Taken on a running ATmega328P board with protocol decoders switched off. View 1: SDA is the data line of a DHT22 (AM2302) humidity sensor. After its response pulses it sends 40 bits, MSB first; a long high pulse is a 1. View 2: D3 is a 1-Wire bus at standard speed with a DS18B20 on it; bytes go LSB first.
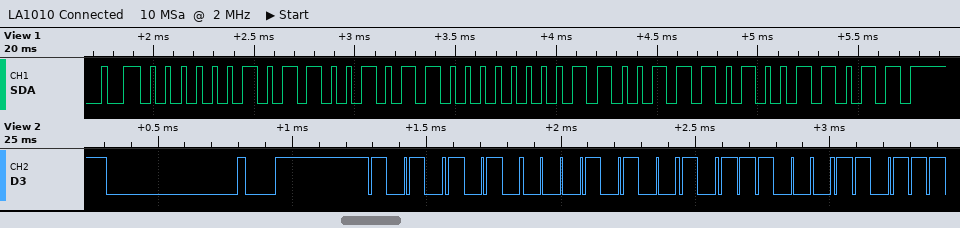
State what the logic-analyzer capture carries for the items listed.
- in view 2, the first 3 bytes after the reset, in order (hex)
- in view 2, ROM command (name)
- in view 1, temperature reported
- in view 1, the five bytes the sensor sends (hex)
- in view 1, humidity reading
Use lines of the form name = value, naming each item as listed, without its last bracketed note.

in view 2, the first 3 bytes after the reset, in order = 55 28 1D
in view 2, ROM command = Match ROM
in view 1, temperature reported = 20.6 °C
in view 1, the five bytes the sensor sends = 02 CB 00 CE 9B
in view 1, humidity reading = 71.5 %
